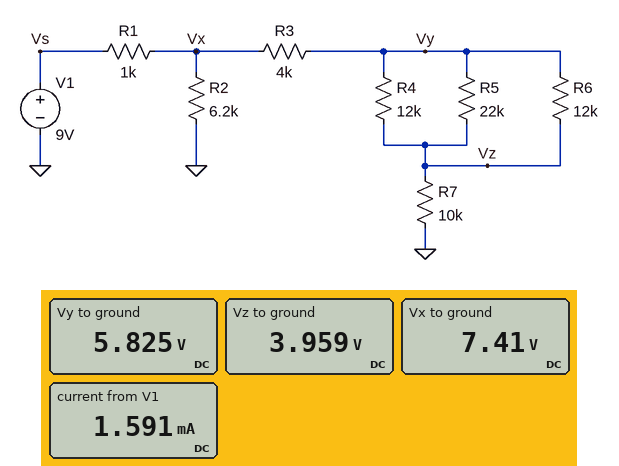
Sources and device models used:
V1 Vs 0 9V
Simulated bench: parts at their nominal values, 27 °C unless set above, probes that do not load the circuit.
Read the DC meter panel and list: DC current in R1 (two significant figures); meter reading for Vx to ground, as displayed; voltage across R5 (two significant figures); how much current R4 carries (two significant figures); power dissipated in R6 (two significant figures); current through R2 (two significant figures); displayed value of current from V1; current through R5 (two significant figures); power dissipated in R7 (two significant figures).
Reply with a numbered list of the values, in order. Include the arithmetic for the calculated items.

1. (9 V - 7.41 V) / 1 kΩ = 1.6 mA
2. 7.41 V
3. 5.825 V - 3.959 V = 1.9 V
4. (5.825 V - 3.959 V) / 12 kΩ = 160 µA
5. (5.825 V - 3.959 V)^2 / 12 kΩ = 290 µW
6. (7.41 V) / 6.2 kΩ = 1.2 mA
7. 1.591 mA
8. (5.825 V - 3.959 V) / 22 kΩ = 85 µA
9. (3.959 V)^2 / 10 kΩ = 1.6 mW
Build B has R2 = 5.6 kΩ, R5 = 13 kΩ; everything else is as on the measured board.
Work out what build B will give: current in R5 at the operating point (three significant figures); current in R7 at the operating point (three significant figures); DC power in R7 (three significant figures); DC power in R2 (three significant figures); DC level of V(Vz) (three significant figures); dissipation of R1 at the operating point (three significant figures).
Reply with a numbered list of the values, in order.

1. 127 µA
2. 403 µA
3. 1.62 mW
4. 9.50 mW
5. 4.03 V
6. 2.91 mW
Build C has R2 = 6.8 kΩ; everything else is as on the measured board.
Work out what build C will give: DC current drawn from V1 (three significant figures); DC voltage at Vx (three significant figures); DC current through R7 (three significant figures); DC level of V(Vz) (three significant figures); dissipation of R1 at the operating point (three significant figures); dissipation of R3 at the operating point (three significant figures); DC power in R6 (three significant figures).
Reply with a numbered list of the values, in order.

1. 1.50 mA
2. 7.50 V
3. 401 µA
4. 4.01 V
5. 2.26 mW
6. 642 µW
7. 297 µW
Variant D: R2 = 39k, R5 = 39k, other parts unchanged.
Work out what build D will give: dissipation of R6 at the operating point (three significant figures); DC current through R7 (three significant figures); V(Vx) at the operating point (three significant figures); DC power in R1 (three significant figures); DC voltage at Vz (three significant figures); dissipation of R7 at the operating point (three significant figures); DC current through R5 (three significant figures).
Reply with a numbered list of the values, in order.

1. 426 µW
2. 435 µA
3. 8.35 V
4. 421 µW
5. 4.35 V
6. 1.89 mW
7. 58.0 µA
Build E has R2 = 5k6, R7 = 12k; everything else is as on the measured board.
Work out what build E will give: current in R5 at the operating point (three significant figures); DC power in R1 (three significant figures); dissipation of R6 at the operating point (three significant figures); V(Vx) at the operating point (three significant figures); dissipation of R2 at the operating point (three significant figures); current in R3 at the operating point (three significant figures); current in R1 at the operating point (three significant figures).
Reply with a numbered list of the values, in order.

1. 75.9 µA
2. 2.77 mW
3. 232 µW
4. 7.34 V
5. 9.61 mW
6. 354 µA
7. 1.66 mA
